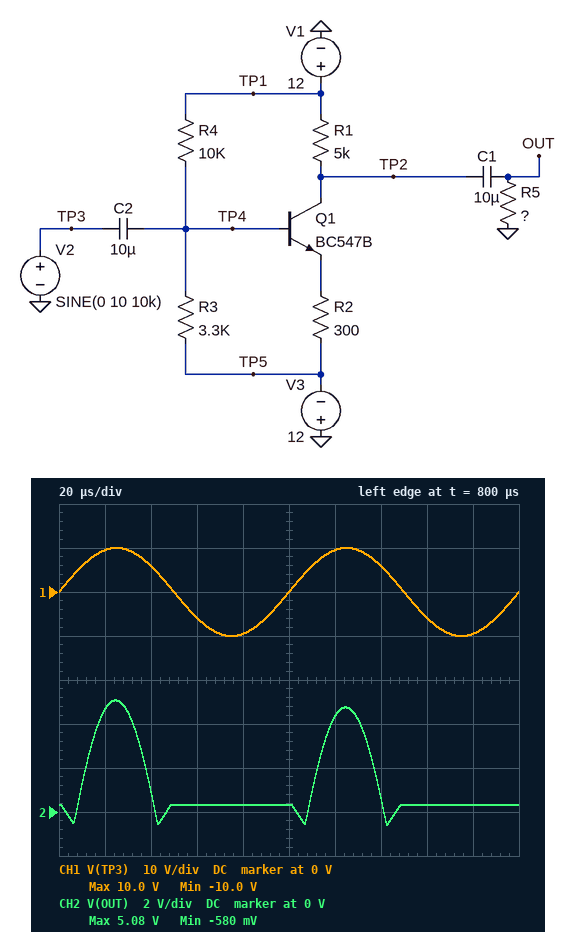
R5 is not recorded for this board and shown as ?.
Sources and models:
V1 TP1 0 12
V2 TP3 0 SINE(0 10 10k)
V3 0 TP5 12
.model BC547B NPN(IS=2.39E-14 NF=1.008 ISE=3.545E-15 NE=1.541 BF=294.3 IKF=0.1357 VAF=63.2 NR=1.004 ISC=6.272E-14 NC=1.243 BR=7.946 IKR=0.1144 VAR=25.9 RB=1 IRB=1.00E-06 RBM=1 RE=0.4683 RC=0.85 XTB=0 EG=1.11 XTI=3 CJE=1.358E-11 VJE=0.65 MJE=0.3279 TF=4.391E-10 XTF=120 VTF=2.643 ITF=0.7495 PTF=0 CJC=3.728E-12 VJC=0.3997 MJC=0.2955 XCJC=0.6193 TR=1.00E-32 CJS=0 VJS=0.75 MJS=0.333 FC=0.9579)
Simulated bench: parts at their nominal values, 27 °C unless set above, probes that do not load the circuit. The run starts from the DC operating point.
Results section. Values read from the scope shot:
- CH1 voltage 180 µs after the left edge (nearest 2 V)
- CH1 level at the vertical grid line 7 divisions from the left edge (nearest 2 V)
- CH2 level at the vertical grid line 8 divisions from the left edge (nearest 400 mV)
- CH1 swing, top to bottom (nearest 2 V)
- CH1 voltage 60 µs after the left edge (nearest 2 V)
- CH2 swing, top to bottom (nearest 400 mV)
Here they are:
-10 V
6 V
400 mV
20 V
-6 V
5.6 V
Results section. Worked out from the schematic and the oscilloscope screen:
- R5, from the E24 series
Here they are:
82 Ω
